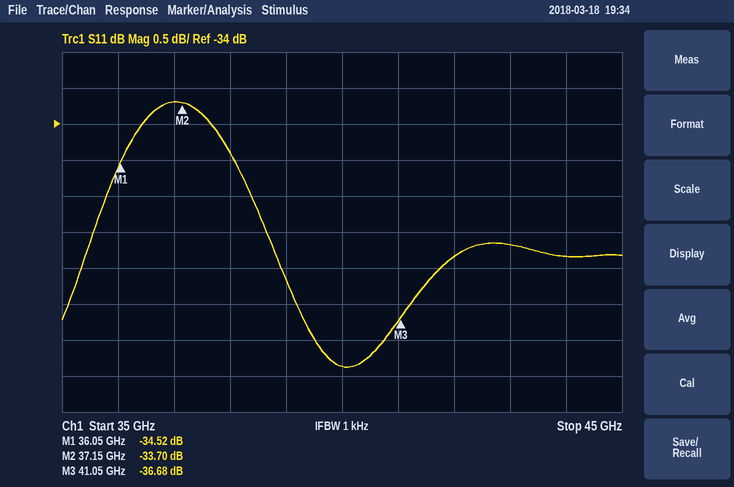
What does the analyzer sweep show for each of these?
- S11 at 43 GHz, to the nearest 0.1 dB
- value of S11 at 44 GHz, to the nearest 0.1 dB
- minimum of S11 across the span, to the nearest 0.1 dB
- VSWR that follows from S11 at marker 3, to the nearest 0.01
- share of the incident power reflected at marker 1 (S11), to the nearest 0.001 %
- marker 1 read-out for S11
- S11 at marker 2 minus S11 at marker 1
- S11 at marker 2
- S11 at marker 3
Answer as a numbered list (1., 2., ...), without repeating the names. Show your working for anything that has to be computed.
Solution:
1. -35.7 dB
2. -35.8 dB
3. -37.4 dB
4. (1 + 0.0147)/(1 − 0.0147) ≈ 1.03
5. 10^(-34.52/10) ≈ 0.035 %
6. -34.52 dB
7. -33.7 − (-34.52) = 0.82 dB
8. -33.70 dB
9. -36.68 dB
